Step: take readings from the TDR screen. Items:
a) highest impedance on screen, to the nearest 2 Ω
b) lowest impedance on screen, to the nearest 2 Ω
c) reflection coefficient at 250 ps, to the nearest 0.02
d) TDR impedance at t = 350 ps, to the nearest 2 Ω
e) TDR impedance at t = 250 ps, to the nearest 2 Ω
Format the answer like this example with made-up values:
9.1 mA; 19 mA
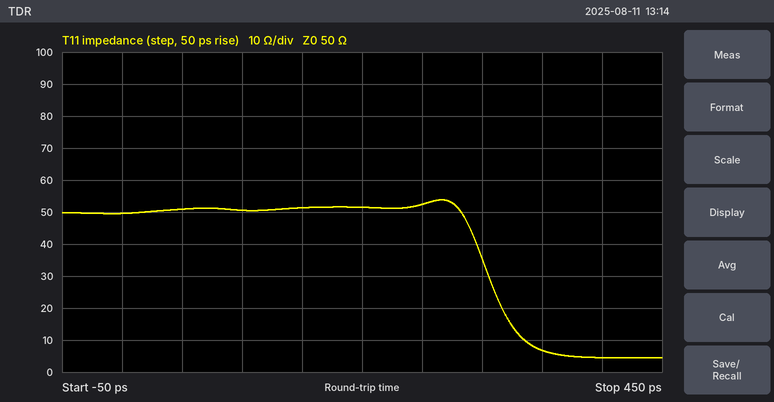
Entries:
54 Ω; 4 Ω; +0.02; 6 Ω; 52 Ω
